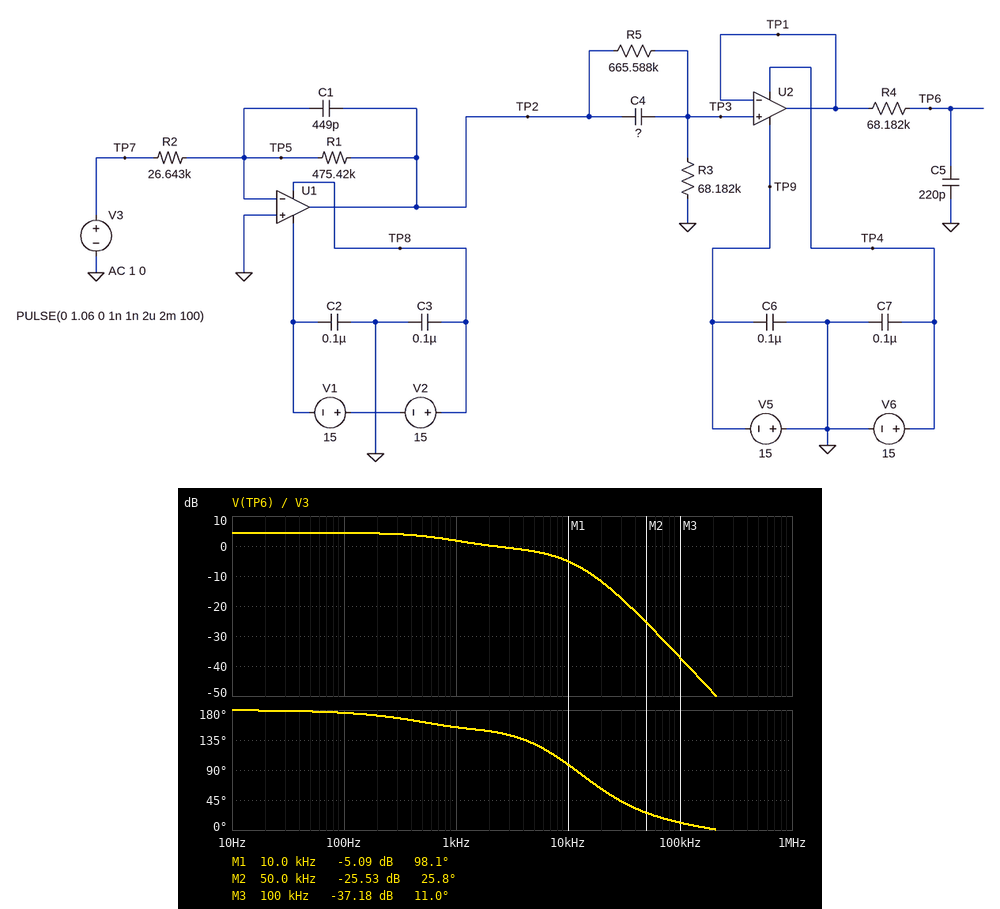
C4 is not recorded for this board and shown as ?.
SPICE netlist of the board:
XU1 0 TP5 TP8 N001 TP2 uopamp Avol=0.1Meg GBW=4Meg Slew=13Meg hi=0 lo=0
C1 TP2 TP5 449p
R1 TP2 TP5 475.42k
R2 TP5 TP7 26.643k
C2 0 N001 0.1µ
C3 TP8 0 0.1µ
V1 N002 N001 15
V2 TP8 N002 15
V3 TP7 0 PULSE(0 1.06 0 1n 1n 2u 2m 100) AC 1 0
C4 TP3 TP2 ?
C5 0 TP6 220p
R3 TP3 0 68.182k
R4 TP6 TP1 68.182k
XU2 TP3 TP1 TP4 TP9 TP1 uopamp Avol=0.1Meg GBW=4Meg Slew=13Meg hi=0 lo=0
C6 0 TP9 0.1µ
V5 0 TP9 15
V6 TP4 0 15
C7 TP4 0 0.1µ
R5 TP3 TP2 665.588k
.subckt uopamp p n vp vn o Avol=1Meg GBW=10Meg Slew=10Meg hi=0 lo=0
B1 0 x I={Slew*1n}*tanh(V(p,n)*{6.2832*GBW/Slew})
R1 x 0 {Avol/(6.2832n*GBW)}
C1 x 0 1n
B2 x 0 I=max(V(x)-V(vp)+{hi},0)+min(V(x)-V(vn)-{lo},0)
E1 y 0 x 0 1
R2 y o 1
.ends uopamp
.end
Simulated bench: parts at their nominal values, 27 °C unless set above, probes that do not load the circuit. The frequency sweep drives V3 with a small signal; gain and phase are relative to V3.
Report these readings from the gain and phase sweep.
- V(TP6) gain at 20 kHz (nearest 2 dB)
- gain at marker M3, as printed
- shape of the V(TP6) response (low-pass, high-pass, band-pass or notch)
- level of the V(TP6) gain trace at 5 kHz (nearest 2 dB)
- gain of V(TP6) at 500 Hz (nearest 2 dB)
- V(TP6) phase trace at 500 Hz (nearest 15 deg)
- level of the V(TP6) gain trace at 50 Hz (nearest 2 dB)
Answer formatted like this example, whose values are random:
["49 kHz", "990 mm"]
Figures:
["-12 dB", "-37.18 dB", "low-pass", "-2 dB", "4 dB", "165 deg", "4 dB"]
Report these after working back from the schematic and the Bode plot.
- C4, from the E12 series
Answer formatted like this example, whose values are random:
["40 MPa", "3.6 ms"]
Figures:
["180 pF"]
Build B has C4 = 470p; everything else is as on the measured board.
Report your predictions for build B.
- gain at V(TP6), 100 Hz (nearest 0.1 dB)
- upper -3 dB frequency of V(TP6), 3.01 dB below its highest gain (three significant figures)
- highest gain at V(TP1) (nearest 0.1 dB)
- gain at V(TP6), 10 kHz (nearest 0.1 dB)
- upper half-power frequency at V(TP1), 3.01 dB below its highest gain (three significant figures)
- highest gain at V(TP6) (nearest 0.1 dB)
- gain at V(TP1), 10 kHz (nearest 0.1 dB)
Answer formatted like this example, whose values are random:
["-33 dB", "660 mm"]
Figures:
["4.5 dB", "5.31 kHz", "6.9 dB", "-1.5 dB", "6.43 kHz", "6.8 dB", "1.3 dB"]
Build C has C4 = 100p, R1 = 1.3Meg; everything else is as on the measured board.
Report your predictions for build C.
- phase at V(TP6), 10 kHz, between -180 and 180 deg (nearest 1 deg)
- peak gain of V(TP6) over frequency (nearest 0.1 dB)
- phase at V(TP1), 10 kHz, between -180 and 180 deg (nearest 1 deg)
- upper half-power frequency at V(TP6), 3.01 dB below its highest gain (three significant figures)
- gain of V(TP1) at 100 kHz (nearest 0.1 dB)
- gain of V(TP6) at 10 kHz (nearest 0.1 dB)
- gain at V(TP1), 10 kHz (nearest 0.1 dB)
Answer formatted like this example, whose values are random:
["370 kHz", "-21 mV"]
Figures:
["103 deg", "13.1 dB", "147 deg", "275 Hz", "-17.8 dB", "-8.9 dB", "-6.1 dB"]
